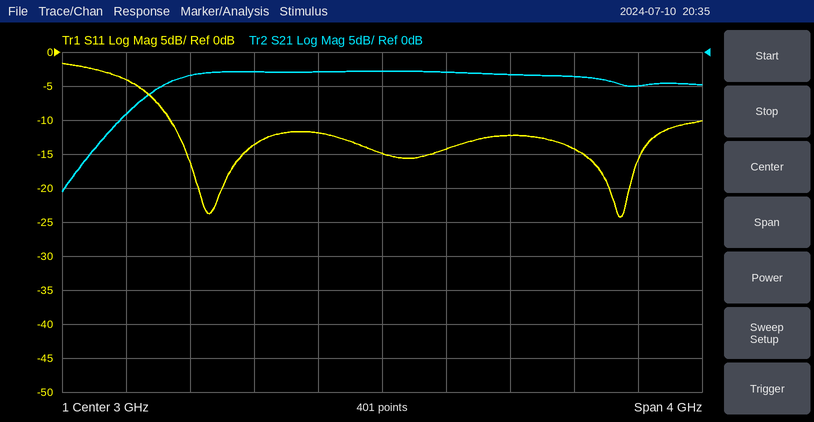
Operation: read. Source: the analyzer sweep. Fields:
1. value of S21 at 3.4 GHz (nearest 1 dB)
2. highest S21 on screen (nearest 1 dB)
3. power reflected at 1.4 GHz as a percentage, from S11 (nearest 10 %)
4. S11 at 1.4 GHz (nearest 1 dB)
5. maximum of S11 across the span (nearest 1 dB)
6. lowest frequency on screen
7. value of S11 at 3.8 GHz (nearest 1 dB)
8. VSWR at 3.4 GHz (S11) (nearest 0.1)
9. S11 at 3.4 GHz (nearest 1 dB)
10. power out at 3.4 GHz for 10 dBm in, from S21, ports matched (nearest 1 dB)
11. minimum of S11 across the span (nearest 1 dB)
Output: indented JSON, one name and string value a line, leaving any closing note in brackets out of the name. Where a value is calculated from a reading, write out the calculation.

{
  "value of S21 at 3.4 GHz": "-3 dB",
  "highest S21 on screen": "-3 dB",
  "power reflected at 1.4 GHz as a percentage, from S11": "10^(-4/10) ≈ 40 %",
  "S11 at 1.4 GHz": "-4 dB",
  "maximum of S11 across the span": "-2 dB",
  "lowest frequency on screen": "1 GHz",
  "value of S11 at 3.8 GHz": "-12 dB",
  "VSWR at 3.4 GHz (S11)": "|Γ| = 10^(-14/20) = 0.1995; VSWR = (1 + 0.1995)/(1 − 0.1995) ≈ 1.5",
  "S11 at 3.4 GHz": "-14 dB",
  "power out at 3.4 GHz for 10 dBm in, from S21, ports matched": "10 dBm + (-3 dB) = 7 dBm",
  "minimum of S11 across the span": "-24 dB"
}
